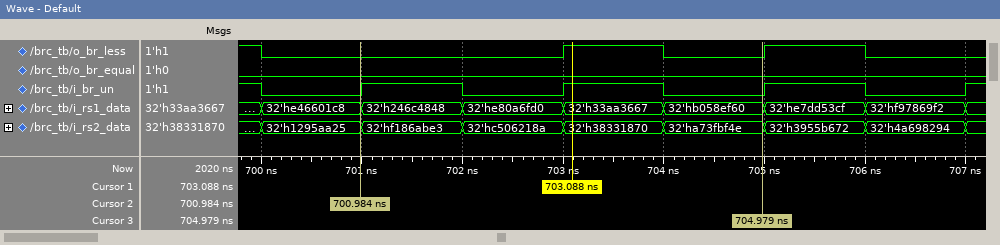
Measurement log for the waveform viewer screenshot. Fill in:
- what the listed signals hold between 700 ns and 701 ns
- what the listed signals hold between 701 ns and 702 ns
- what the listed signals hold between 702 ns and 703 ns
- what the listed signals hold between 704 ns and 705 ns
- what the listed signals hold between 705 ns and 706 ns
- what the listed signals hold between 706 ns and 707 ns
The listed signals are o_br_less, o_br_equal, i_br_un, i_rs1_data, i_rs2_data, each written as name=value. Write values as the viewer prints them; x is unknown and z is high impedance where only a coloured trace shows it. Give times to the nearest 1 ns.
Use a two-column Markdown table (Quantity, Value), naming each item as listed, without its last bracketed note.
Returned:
| Quantity | Value |
|---|---|
| what the listed signals hold between 700 ns and 701 ns | o_br_less=0, o_br_equal=0, i_br_un=0, i_rs1_data=32'he46601c8, i_rs2_data=32'h1295aa25 |
| what the listed signals hold between 701 ns and 702 ns | o_br_less=0, o_br_equal=0, i_br_un=1, i_rs1_data=32'h246c4848, i_rs2_data=32'hf186abe3 |
| what the listed signals hold between 702 ns and 703 ns | o_br_less=0, o_br_equal=0, i_br_un=0, i_rs1_data=32'he80a6fd0, i_rs2_data=32'hc506218a |
| what the listed signals hold between 704 ns and 705 ns | o_br_less=0, o_br_equal=0, i_br_un=0, i_rs1_data=32'hb058ef60, i_rs2_data=32'ha73fbf4e |
| what the listed signals hold between 705 ns and 706 ns | o_br_less=1, o_br_equal=0, i_br_un=1, i_rs1_data=32'he7dd53cf, i_rs2_data=32'h3955b672 |
| what the listed signals hold between 706 ns and 707 ns | o_br_less=0, o_br_equal=0, i_br_un=0, i_rs1_data=32'hf97869f2, i_rs2_data=32'h4a698294 |
